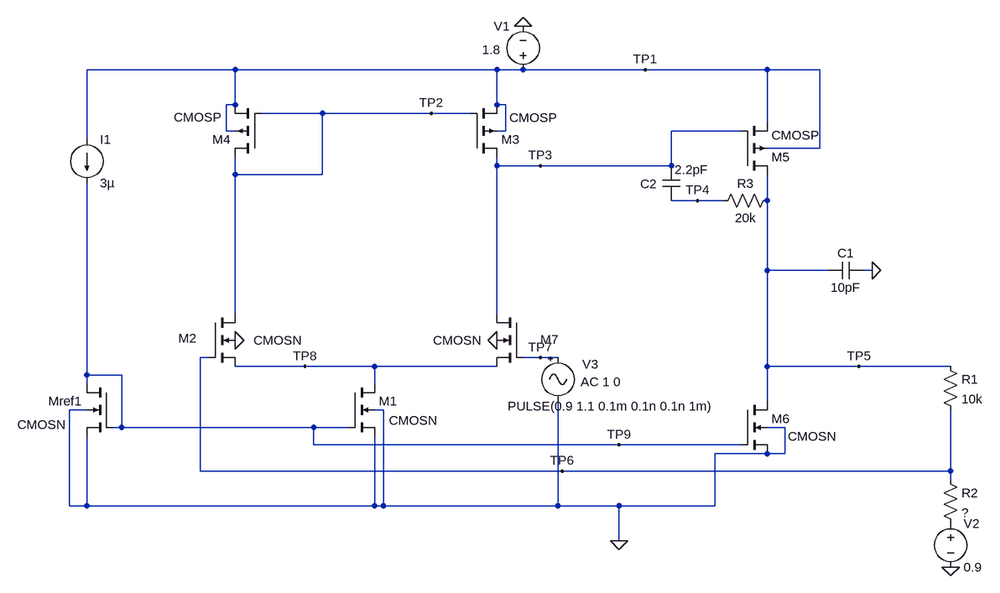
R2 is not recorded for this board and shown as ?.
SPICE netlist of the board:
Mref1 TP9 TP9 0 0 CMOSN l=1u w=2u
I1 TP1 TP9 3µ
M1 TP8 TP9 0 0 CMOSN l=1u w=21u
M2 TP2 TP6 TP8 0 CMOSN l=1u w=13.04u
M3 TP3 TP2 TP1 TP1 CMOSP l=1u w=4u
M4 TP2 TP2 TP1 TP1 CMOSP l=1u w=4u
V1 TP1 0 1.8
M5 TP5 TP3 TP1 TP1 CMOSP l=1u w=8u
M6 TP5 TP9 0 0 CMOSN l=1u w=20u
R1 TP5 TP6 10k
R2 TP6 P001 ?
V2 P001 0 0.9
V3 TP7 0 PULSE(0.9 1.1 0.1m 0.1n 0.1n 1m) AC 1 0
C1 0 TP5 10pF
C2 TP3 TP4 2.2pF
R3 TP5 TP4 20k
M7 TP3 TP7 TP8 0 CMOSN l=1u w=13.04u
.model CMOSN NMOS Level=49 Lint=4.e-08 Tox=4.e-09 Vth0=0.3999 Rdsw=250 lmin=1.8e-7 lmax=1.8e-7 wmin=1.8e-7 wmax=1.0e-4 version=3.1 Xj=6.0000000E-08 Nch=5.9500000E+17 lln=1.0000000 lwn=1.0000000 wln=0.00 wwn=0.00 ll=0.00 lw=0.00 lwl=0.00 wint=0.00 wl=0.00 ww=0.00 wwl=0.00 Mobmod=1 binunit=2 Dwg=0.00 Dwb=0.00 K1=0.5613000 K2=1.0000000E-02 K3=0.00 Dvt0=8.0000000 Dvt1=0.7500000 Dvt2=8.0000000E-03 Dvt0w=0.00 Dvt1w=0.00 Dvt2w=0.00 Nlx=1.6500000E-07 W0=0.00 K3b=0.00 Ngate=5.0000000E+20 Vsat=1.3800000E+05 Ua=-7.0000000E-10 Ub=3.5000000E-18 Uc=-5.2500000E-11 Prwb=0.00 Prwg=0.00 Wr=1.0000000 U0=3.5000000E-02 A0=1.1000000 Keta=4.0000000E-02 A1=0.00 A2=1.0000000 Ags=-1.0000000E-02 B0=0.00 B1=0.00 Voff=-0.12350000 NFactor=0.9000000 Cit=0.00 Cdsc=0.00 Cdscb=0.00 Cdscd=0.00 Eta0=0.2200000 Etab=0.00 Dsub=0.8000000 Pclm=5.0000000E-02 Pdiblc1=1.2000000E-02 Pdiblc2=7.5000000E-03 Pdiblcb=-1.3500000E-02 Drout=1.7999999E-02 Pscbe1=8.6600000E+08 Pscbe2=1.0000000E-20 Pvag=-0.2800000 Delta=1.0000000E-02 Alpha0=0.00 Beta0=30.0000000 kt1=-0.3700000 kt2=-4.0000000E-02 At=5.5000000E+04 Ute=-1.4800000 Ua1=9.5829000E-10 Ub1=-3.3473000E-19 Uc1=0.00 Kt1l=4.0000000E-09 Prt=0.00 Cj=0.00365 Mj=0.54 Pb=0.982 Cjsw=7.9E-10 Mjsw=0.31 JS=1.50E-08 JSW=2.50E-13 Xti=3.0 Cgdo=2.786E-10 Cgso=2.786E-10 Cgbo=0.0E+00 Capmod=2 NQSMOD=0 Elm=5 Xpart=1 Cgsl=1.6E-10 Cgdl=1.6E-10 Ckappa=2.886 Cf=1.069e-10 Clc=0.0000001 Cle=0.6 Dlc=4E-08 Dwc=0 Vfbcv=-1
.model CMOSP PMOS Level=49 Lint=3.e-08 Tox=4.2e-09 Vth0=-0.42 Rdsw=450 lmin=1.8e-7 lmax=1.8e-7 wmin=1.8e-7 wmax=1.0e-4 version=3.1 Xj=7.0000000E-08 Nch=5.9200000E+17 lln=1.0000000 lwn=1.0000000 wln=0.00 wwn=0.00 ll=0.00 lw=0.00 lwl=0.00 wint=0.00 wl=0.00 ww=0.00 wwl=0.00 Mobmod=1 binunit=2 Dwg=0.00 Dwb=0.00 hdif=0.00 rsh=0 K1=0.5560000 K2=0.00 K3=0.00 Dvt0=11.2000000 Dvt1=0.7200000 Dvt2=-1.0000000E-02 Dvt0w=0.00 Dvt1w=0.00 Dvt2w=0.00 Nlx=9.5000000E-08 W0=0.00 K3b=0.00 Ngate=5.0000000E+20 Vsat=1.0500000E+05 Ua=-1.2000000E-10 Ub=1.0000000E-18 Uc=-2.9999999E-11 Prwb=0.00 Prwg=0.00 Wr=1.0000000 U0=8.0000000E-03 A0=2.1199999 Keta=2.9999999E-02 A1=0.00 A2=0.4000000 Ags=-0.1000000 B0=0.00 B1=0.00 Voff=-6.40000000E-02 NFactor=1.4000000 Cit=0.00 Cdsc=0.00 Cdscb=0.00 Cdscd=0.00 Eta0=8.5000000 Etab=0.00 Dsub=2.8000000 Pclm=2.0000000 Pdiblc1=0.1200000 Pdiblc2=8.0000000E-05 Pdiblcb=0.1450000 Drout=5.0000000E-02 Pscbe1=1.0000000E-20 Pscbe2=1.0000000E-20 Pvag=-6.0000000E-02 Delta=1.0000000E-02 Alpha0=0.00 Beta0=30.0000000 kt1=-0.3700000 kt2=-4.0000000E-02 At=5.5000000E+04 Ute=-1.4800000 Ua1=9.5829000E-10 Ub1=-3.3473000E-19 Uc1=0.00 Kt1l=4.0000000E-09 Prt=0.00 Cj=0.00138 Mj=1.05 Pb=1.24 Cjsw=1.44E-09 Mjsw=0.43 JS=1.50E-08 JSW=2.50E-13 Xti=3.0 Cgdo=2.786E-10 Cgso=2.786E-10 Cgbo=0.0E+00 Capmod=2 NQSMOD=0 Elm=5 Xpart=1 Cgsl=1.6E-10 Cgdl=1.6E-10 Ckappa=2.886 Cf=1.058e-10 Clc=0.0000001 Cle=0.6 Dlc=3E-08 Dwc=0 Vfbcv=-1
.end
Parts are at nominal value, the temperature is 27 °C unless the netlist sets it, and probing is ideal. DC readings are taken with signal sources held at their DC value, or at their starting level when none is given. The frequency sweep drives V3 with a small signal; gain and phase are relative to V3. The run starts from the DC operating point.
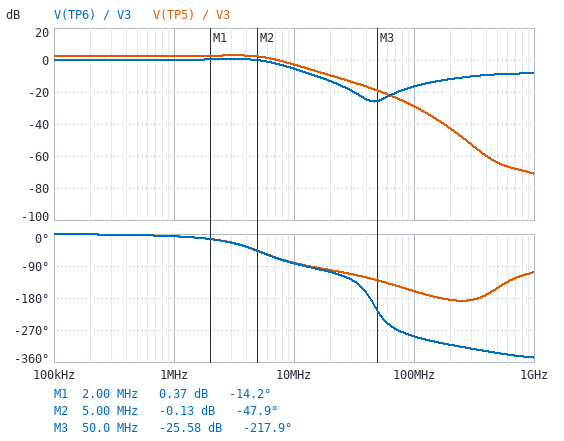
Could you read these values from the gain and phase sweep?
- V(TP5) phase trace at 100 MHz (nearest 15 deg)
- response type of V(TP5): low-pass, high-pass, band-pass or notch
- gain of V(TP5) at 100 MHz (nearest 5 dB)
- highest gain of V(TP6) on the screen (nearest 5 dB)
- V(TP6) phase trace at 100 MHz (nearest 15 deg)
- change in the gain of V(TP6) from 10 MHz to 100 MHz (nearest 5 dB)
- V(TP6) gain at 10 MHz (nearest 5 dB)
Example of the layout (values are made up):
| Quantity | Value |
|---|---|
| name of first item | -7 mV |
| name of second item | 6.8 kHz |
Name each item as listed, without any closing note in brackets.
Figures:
| Quantity | Value |
|---|---|
| V(TP5) phase trace at 100 MHz | -165 deg |
| response type of V(TP5): low-pass, high-pass, band-pass or notch | low-pass |
| gain of V(TP5) at 100 MHz | -30 dB |
| highest gain of V(TP6) on the screen | 0 dB |
| V(TP6) phase trace at 100 MHz | -285 deg |
| change in the gain of V(TP6) from 10 MHz to 100 MHz | -10 dB |
| V(TP6) gain at 10 MHz | -5 dB |
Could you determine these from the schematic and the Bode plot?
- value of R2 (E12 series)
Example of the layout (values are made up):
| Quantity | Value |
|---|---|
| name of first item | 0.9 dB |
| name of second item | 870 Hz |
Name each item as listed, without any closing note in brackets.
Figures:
| Quantity | Value |
|---|---|
| value of R2 | 33 kΩ |
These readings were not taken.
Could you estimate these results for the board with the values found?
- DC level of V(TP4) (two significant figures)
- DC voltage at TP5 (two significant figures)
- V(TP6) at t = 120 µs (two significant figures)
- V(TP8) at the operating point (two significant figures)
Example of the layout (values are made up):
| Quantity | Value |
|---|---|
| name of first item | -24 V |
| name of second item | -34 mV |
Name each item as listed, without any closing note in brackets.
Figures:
| Quantity | Value |
|---|---|
| DC level of V(TP4) | 900 mV |
| DC voltage at TP5 | 900 mV |
| V(TP6) at t = 120 µs | 1.1 V |
| V(TP8) at the operating point | 310 mV |
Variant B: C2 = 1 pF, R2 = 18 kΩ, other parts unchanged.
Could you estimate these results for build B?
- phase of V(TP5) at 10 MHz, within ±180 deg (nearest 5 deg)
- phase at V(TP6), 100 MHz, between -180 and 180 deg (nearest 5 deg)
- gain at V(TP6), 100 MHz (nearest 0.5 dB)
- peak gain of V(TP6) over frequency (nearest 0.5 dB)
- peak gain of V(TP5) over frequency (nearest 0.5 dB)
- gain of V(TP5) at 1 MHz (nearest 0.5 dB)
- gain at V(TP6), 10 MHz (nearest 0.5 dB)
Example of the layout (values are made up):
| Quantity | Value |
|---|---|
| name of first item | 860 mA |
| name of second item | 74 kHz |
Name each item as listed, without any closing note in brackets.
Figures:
| Quantity | Value |
|---|---|
| phase of V(TP5) at 10 MHz, within ±180 deg | -95 deg |
| phase at V(TP6), 100 MHz, between -180 and 180 deg | 75 deg |
| gain at V(TP6), 100 MHz | -18.0 dB |
| peak gain of V(TP6) over frequency | 2.5 dB |
| peak gain of V(TP5) over frequency | 6.0 dB |
| gain of V(TP5) at 1 MHz | 4.0 dB |
| gain at V(TP6), 10 MHz | -2.5 dB |
